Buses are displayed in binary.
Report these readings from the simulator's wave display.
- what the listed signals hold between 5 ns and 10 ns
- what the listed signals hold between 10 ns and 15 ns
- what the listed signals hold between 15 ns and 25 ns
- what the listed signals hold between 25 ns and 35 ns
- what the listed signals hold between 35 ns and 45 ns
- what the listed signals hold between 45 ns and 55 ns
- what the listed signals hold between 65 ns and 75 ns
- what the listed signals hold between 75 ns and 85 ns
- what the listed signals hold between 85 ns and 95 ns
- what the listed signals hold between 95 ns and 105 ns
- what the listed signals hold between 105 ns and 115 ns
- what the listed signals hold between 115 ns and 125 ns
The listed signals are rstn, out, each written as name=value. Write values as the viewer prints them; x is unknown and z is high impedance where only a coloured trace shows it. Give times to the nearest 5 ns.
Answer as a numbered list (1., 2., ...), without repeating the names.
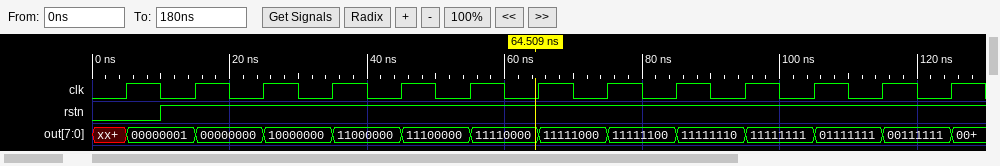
1. rstn=0, out=00000001
2. rstn=1, out=00000001
3. rstn=1, out=00000000
4. rstn=1, out=10000000
5. rstn=1, out=11000000
6. rstn=1, out=11100000
7. rstn=1, out=11111000
8. rstn=1, out=11111100
9. rstn=1, out=11111110
10. rstn=1, out=11111111
11. rstn=1, out=01111111
12. rstn=1, out=00111111
